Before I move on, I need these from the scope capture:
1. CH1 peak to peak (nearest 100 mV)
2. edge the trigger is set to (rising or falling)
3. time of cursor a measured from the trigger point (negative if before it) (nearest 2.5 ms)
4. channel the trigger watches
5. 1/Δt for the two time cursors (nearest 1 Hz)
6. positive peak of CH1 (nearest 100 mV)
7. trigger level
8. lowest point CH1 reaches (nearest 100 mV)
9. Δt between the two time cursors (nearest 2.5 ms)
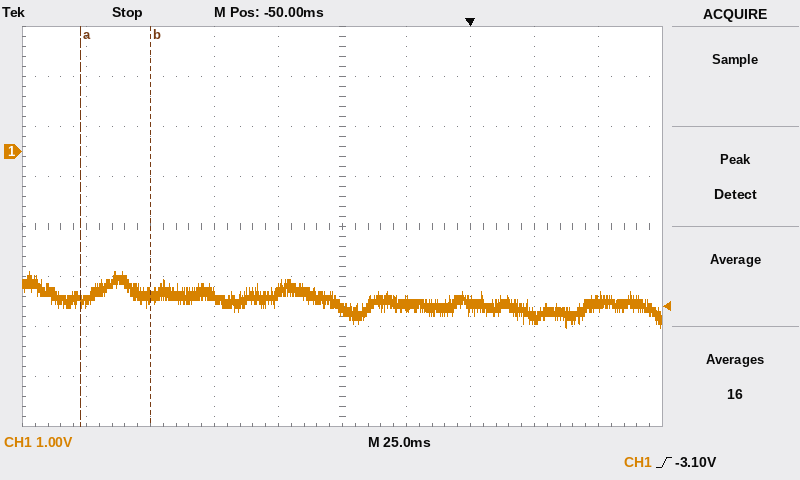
1.1 V
rising
-152.5 ms
CH1
36 Hz
-2.4 V
-3.10 V
-3.5 V
27.5 ms
